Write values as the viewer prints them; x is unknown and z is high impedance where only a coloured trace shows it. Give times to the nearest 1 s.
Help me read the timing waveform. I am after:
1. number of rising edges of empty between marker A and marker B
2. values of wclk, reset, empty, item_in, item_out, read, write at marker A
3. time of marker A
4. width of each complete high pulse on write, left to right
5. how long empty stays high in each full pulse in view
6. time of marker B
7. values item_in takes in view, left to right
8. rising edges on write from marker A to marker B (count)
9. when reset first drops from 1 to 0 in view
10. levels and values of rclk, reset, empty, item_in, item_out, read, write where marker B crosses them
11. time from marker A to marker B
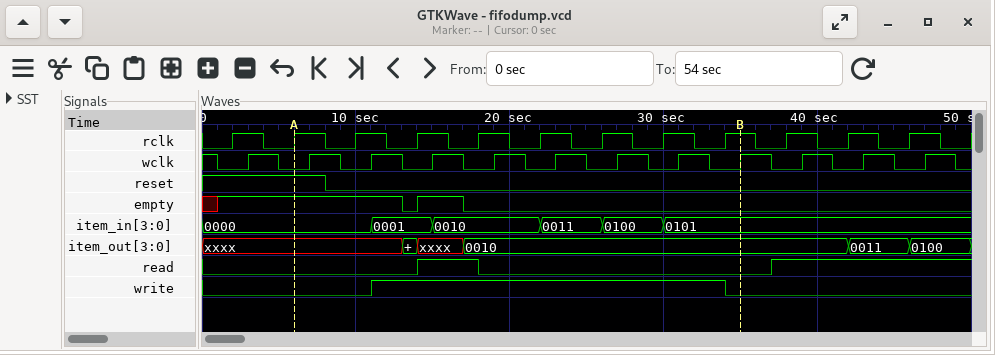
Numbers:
1
wclk=0, reset=1, empty=1, item_in=0000, item_out=xxxx, read=0, write=0
6 s
23 s
3 s
35 s
0000, 0001, 0010, 0011, 0100, 0101
1
8 s
rclk=1, reset=0, empty=0, item_in=0101, item_out=0010, read=0, write=0
29 s
